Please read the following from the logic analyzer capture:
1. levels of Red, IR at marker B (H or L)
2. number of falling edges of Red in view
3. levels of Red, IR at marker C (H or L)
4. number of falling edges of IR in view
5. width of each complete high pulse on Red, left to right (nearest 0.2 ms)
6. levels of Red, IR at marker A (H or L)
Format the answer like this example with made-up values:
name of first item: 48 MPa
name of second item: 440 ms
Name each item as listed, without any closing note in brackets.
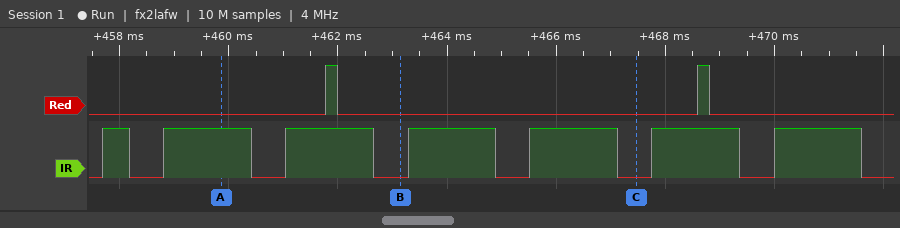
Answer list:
levels of Red, IR at marker B: Red=L, IR=L
number of falling edges of Red in view: 2
levels of Red, IR at marker C: Red=L, IR=L
number of falling edges of IR in view: 7
width of each complete high pulse on Red, left to right: 0.2 ms, 0.2 ms
levels of Red, IR at marker A: Red=L, IR=H
